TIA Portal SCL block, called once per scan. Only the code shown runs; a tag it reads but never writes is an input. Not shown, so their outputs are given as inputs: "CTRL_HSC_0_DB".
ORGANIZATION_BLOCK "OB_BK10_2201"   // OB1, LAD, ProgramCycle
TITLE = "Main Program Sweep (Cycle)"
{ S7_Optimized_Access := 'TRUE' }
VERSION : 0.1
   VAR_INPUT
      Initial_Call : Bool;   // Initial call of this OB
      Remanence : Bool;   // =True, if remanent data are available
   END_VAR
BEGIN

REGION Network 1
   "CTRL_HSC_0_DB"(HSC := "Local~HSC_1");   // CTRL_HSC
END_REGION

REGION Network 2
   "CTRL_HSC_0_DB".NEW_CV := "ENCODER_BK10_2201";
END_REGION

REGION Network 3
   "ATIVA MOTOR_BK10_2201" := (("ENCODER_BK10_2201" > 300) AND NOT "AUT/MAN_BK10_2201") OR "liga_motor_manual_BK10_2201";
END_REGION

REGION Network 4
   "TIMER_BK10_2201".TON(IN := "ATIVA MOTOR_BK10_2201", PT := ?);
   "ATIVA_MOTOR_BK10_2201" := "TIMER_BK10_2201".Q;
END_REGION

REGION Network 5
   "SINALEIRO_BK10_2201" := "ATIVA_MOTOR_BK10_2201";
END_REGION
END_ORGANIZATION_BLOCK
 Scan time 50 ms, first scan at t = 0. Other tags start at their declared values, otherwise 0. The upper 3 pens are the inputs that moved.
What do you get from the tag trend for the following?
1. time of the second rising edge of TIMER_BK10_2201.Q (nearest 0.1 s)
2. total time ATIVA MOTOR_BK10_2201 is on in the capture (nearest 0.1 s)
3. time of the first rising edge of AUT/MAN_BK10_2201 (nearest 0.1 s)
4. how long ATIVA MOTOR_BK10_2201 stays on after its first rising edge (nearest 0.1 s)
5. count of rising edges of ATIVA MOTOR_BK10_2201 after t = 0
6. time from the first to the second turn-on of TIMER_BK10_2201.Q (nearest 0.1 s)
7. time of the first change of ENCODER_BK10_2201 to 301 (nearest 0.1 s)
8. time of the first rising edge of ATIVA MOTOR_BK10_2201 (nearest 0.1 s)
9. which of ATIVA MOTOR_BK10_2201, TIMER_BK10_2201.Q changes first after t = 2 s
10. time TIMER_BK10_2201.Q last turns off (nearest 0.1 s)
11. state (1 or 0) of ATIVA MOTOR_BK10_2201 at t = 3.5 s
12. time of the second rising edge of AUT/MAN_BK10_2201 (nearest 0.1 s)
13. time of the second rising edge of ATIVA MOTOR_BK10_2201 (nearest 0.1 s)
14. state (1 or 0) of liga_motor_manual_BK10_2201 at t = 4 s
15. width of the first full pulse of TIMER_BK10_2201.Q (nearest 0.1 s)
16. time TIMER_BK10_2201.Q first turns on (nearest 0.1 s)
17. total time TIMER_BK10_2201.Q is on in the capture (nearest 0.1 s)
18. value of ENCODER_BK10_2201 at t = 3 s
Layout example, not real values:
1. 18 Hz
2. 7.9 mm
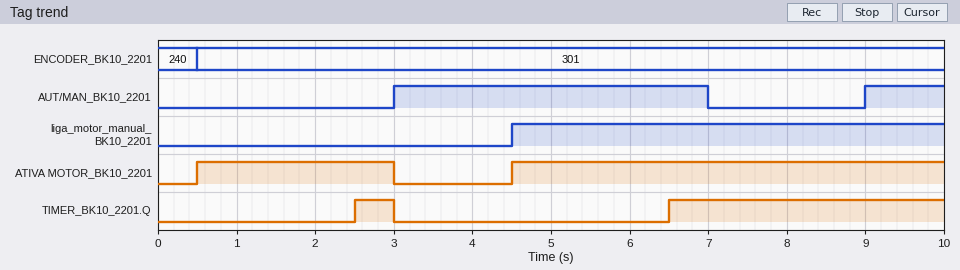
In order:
1. 6.5 s
2. 8.0 s
3. 3.0 s
4. 2.5 s
5. 2
6. 4.0 s
7. 0.5 s
8. 0.5 s
9. TIMER_BK10_2201.Q
10. 3.0 s
11. 0
12. 9.0 s
13. 4.5 s
14. 0
15. 0.5 s
16. 2.5 s
17. 4.0 s
18. 301
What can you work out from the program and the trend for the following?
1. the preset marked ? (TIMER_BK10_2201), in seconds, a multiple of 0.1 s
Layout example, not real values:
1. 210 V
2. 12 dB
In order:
1. 2.0 s
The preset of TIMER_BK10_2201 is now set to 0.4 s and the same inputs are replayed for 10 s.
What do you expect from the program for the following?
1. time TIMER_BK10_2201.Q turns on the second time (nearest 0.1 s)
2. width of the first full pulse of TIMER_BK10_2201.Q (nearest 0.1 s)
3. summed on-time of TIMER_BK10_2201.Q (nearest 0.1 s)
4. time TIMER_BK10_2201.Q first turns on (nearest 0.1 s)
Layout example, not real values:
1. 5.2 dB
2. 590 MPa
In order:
1. 4.9 s
2. 2.1 s
3. 7.2 s
4. 0.9 s
